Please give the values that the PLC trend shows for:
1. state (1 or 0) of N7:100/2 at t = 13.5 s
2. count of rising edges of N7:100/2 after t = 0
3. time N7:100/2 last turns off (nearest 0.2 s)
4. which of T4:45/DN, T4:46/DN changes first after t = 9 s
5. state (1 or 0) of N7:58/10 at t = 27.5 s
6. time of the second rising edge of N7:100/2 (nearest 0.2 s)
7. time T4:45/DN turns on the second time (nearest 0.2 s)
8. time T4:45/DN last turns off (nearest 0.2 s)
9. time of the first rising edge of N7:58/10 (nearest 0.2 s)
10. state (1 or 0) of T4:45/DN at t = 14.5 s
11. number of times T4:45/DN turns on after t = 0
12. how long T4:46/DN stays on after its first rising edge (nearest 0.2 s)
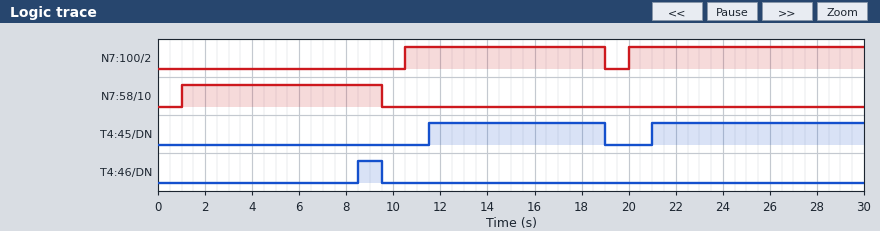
1
2
19.0 s
T4:46/DN
0
20.0 s
21.0 s
19.0 s
1.0 s
1
2
1.0 s
